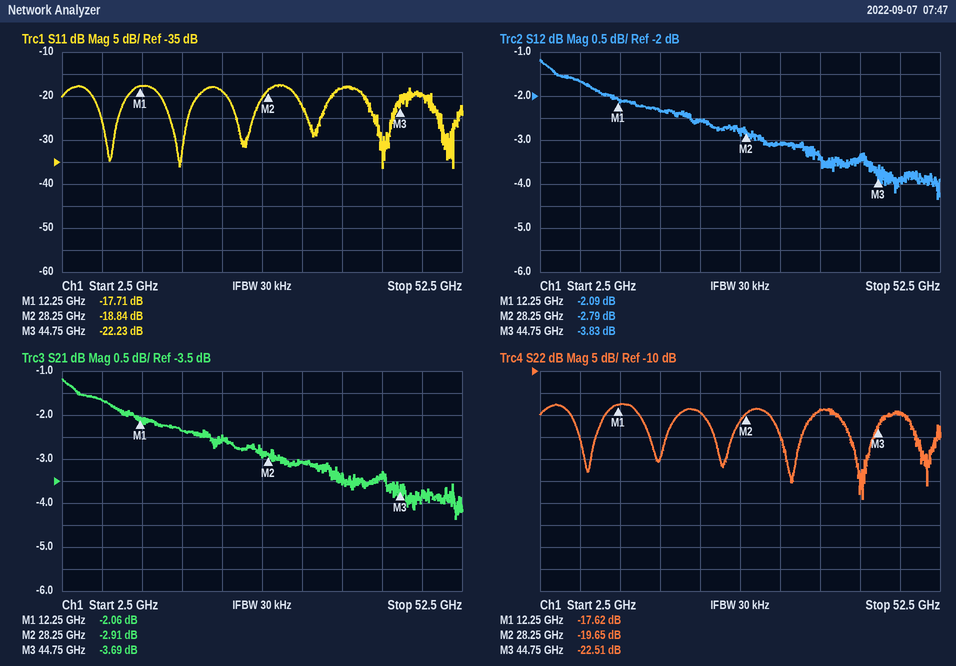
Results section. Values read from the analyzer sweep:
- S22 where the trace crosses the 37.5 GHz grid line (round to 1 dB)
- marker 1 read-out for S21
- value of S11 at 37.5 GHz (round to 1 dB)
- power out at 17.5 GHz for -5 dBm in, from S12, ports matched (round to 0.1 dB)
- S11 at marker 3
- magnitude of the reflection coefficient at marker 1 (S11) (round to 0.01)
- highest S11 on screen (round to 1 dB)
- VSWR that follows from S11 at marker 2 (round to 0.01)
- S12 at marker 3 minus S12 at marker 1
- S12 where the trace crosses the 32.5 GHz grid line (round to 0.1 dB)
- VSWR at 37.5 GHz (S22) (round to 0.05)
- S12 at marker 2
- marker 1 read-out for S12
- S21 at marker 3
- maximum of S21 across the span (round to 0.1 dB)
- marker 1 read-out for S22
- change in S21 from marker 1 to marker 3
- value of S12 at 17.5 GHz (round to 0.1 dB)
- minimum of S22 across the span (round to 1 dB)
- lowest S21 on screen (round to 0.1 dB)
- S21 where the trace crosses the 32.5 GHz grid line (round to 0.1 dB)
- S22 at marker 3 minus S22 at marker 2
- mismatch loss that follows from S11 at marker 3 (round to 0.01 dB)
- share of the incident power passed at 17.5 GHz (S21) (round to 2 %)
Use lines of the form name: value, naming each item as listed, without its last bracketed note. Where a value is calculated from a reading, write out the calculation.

S22 where the trace crosses the 37.5 GHz grid line: -19 dB
marker 1 read-out for S21: -2.06 dB
value of S11 at 37.5 GHz: -18 dB
power out at 17.5 GHz for -5 dBm in, from S12, ports matched: -5 dBm + (-2.3 dB) = -7.3 dBm
S11 at marker 3: -22.23 dB
magnitude of the reflection coefficient at marker 1 (S11): 10^(-17.71/20) ≈ 0.13
highest S11 on screen: -17 dB
VSWR that follows from S11 at marker 2: (1 + 0.1143)/(1 − 0.1143) ≈ 1.26
S12 at marker 3 minus S12 at marker 1: -3.83 − (-2.09) = -1.74 dB
S12 where the trace crosses the 32.5 GHz grid line: -3.1 dB
VSWR at 37.5 GHz (S22): |Γ| = 10^(-19/20) = 0.1122; VSWR = (1 + 0.1122)/(1 − 0.1122) ≈ 1.25
S12 at marker 2: -2.79 dB
marker 1 read-out for S12: -2.09 dB
S21 at marker 3: -3.69 dB
maximum of S21 across the span: -1.2 dB
marker 1 read-out for S22: -17.62 dB
change in S21 from marker 1 to marker 3: -3.69 − (-2.06) = -1.63 dB
value of S12 at 17.5 GHz: -2.3 dB
minimum of S22 across the span: -39 dB
lowest S21 on screen: -4.4 dB
S21 where the trace crosses the 32.5 GHz grid line: -3.1 dB
S22 at marker 3 minus S22 at marker 2: -22.51 − (-19.65) = -2.86 dB
mismatch loss that follows from S11 at marker 3: −10 log10(1 − 10^(-22.23/10)) ≈ 0.03 dB
share of the incident power passed at 17.5 GHz (S21): 10^(-2.4/10) ≈ 58 %
